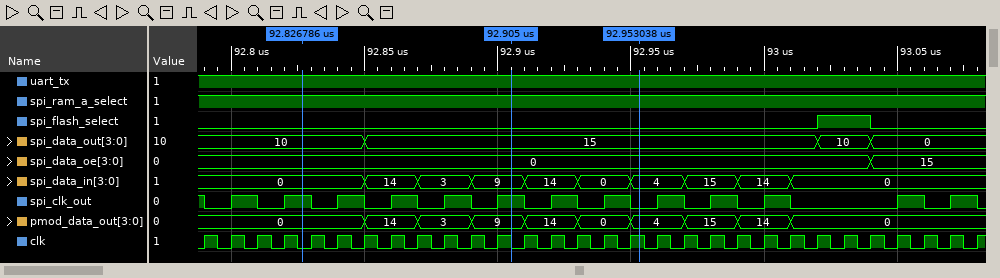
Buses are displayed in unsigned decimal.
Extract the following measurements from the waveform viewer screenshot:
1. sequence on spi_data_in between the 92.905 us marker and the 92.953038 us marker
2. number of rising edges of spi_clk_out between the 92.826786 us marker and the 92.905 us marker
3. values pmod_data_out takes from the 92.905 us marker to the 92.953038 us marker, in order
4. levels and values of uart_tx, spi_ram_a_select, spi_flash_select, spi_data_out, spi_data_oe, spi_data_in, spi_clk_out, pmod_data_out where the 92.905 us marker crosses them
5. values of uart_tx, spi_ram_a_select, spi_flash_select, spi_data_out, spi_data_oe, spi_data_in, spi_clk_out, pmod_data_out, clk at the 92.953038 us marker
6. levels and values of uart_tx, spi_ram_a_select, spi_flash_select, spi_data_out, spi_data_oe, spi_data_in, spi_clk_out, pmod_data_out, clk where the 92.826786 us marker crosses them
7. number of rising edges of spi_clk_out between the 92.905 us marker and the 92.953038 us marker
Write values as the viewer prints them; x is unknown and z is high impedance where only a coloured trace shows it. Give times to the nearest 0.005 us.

9, 14, 0, 4
4
9, 14, 0, 4
uart_tx=1, spi_ram_a_select=1, spi_flash_select=0, spi_data_out=15, spi_data_oe=0, spi_data_in=9, spi_clk_out=1, pmod_data_out=9
uart_tx=1, spi_ram_a_select=1, spi_flash_select=0, spi_data_out=15, spi_data_oe=0, spi_data_in=4, spi_clk_out=0, pmod_data_out=4, clk=1
uart_tx=1, spi_ram_a_select=1, spi_flash_select=0, spi_data_out=10, spi_data_oe=0, spi_data_in=0, spi_clk_out=1, pmod_data_out=0, clk=0
2
